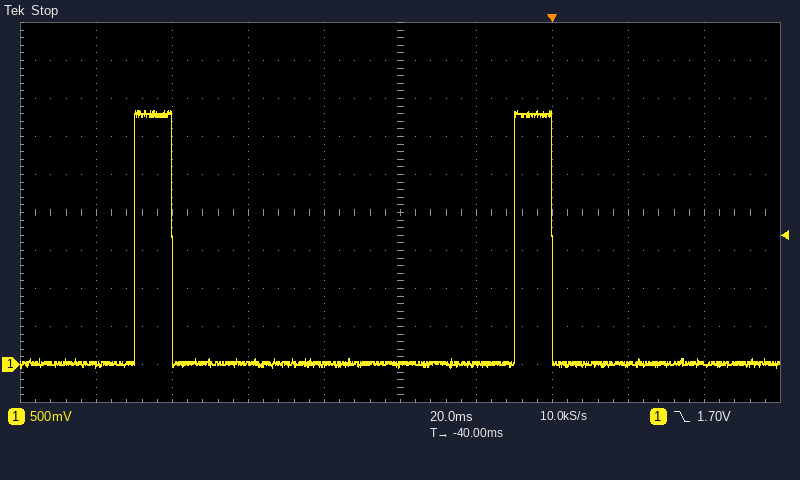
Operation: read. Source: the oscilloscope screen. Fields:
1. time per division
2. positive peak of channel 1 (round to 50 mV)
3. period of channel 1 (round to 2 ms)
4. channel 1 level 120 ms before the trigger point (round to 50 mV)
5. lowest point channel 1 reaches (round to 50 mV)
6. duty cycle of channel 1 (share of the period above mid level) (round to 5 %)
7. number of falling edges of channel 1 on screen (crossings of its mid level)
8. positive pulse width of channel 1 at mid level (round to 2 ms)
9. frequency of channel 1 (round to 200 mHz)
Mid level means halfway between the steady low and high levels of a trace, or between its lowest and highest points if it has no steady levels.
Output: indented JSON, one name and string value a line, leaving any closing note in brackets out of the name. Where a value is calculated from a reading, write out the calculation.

{
  "time per division": "20 ms",
  "positive peak of channel 1": "3.35 V",
  "period of channel 1": "100 ms",
  "channel 1 level 120 ms before the trigger point": "0 mV",
  "lowest point channel 1 reaches": "-50 mV",
  "duty cycle of channel 1 (share of the period above mid level)": "10 ms / 100 ms ≈ 10 %",
  "number of falling edges of channel 1 on screen": "2",
  "positive pulse width of channel 1 at mid level": "10 ms",
  "frequency of channel 1": "1 / 100 ms ≈ 10.0 Hz"
}
